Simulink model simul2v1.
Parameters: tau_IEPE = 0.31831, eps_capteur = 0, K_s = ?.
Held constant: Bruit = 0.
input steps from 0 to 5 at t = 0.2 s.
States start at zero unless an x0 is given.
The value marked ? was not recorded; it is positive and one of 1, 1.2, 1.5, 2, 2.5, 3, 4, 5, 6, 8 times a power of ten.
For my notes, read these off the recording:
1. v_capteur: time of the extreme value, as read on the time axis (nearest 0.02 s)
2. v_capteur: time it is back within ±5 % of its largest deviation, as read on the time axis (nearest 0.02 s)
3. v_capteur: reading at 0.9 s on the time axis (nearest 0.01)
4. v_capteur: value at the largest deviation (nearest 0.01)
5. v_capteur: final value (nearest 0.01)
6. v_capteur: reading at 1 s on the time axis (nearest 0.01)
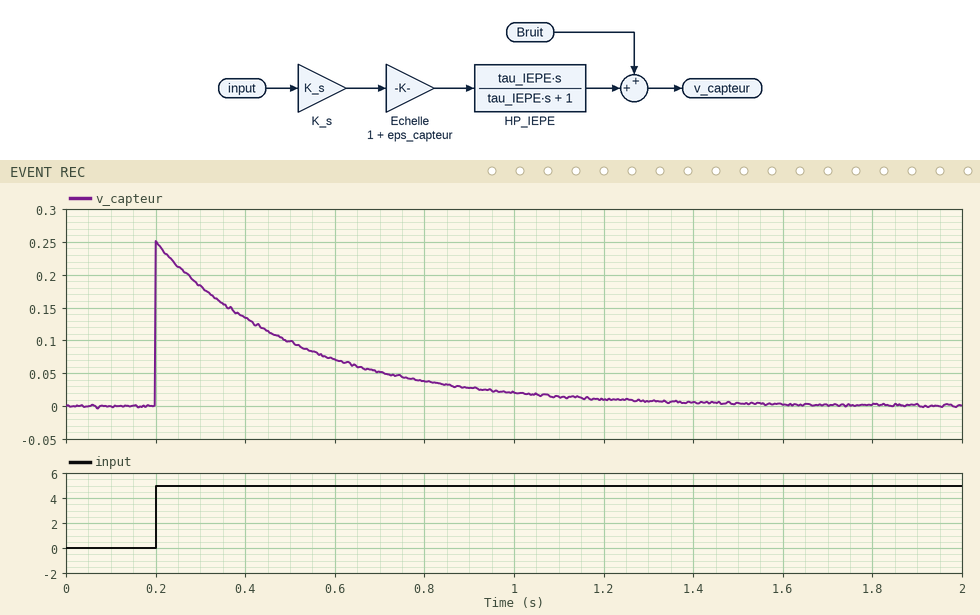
0.20 s
1.16 s
0.03
0.25
0.00
0.02
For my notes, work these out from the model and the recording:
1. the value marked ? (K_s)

0.05
